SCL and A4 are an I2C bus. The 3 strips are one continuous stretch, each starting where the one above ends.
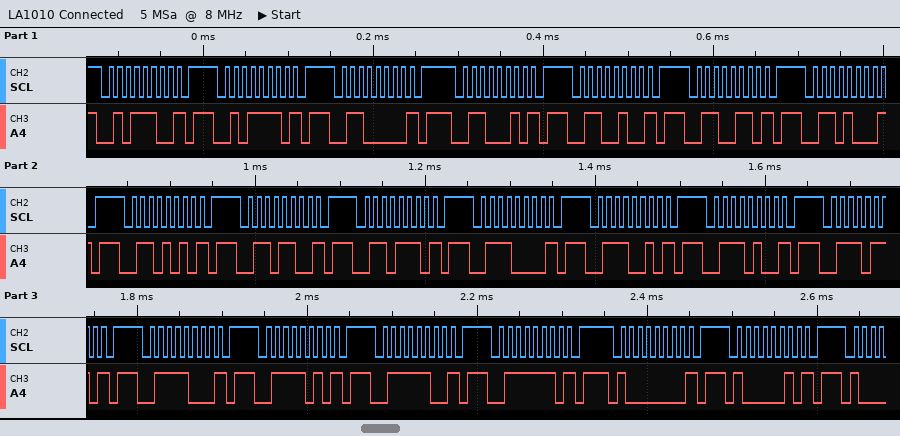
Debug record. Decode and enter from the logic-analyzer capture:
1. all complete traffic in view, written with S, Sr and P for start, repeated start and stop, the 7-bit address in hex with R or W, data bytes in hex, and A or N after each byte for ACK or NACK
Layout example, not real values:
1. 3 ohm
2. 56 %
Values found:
1. S 2EW N P S 2FW N P S 30W N P S 31W N P S 32W N P S 33W N P S 34W N P S 35W N P S 36W N P S 37W N P S 38W N P S 39W N P S 3AW N P S 3BW N P S 3CW N P S 3DW N P S 3EW N P S 3FW N P S 40W N P S 41W N P
